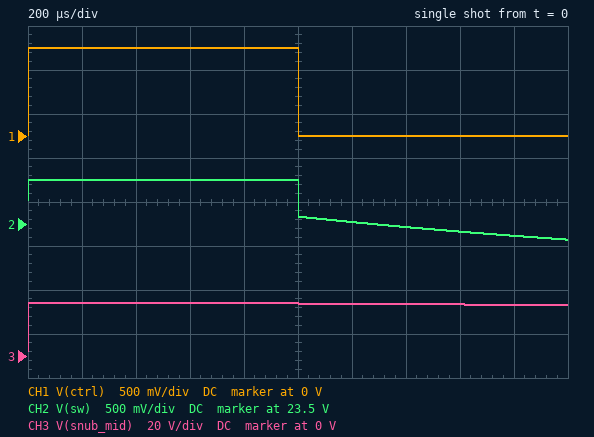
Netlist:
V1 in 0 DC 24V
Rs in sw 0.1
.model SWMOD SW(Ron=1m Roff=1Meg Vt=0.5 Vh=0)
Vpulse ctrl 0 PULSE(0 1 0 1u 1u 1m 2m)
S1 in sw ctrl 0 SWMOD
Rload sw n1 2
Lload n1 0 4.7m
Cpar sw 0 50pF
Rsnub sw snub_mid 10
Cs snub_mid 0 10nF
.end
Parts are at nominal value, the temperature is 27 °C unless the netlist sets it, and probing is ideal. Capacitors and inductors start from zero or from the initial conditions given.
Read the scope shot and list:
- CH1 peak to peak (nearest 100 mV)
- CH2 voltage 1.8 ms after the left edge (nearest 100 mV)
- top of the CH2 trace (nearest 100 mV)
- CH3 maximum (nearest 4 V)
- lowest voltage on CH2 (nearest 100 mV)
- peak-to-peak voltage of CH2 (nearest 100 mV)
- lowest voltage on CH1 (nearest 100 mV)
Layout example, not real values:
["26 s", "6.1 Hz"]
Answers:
["1.0 V", "23.4 V", "24.0 V", "24 V", "23.3 V", "700 mV", "0 V"]
